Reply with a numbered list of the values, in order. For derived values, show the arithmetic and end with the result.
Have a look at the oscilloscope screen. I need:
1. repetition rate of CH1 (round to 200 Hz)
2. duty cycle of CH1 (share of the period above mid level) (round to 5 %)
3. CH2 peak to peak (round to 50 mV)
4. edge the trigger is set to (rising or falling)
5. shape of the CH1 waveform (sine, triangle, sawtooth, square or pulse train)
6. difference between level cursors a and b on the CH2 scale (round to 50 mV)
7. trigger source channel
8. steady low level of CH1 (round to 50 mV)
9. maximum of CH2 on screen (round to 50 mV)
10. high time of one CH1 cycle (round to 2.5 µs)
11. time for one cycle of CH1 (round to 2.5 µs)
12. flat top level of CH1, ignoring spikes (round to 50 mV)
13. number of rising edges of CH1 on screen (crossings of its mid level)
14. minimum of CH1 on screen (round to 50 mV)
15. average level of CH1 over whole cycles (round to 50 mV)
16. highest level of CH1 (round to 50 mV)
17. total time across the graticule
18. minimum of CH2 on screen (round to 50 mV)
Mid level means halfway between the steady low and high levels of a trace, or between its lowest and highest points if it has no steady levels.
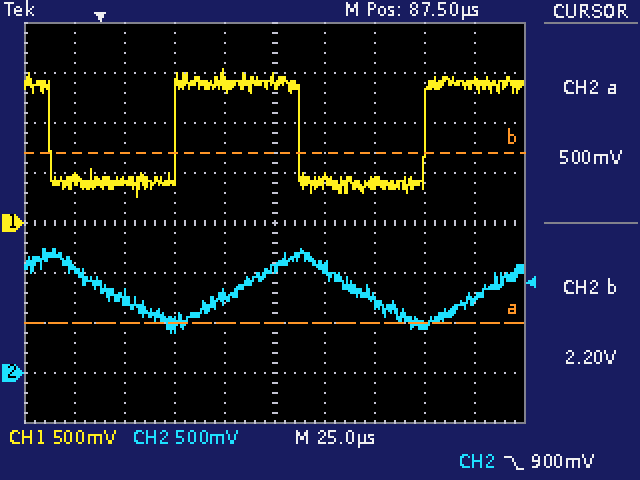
1. 1 / 125.0 µs ≈ 8.0 kHz
2. 62.5 µs / 125.0 µs ≈ 50 %
3. 1.25 V − (400 mV) = 850 mV
4. falling
5. square
6. 1.70 V
7. CH2
8. 400 mV
9. 1.25 V
10. 62.5 µs
11. 125.0 µs
12. 1.40 V
13. 2
14. 250 mV
15. 400 mV + 0.5 × (1.40 V − (400 mV)) ≈ 900 mV
16. 1.55 V
17. 250 µs
18. 400 mV
